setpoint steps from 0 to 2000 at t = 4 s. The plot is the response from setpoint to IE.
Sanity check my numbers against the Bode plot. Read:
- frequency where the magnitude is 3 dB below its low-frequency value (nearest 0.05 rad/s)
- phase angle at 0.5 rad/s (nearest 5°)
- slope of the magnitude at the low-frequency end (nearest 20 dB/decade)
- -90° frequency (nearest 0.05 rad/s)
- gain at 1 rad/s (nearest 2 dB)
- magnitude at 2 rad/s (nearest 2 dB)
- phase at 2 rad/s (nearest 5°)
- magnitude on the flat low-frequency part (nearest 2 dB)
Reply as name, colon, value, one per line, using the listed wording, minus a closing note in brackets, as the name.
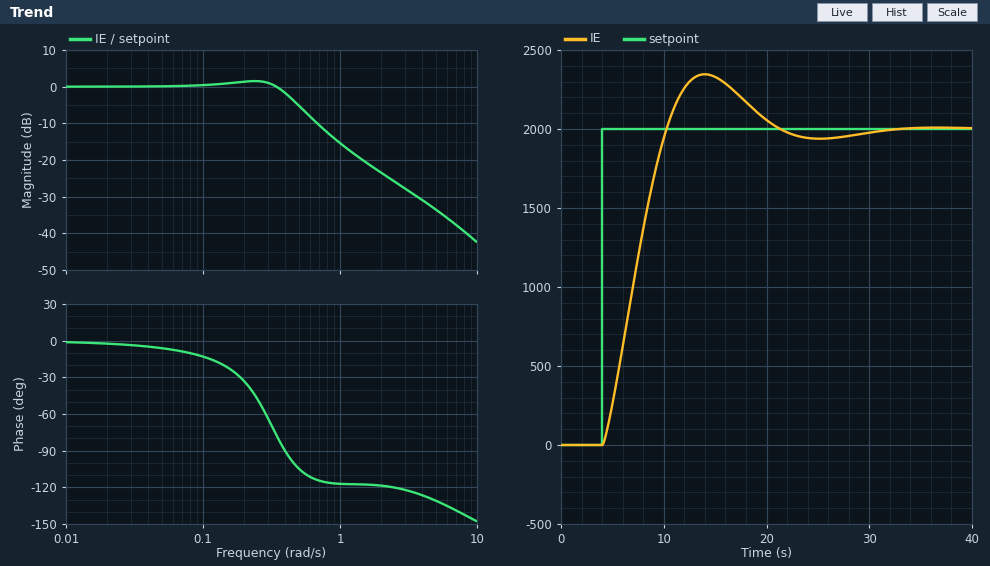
frequency where the magnitude is 3 dB below its low-frequency value: 0.45 rad/s
phase angle at 0.5 rad/s: -105°
slope of the magnitude at the low-frequency end: 0 dB/decade
-90° frequency: 0.40 rad/s
gain at 1 rad/s: -16 dB
magnitude at 2 rad/s: -24 dB
phase at 2 rad/s: -120°
magnitude on the flat low-frequency part: 0 dB
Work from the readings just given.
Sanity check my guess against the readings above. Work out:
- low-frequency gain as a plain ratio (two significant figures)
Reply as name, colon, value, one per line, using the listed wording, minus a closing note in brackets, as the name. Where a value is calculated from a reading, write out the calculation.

low-frequency gain as a plain ratio: 10^(0 / 20) = 1.0
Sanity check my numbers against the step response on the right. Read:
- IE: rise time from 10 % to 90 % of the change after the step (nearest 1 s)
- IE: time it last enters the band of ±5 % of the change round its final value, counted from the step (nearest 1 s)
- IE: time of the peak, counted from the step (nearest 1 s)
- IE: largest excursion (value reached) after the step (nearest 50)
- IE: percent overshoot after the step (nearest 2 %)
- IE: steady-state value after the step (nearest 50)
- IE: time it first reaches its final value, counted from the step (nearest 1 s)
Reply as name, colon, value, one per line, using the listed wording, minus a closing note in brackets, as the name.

IE: rise time from 10 % to 90 % of the change after the step: 5 s
IE: time it last enters the band of ±5 % of the change round its final value, counted from the step: 15 s
IE: time of the peak, counted from the step: 10 s
IE: largest excursion (value reached) after the step: 2350
IE: percent overshoot after the step: 18 %
IE: steady-state value after the step: 2000
IE: time it first reaches its final value, counted from the step: 6 s
